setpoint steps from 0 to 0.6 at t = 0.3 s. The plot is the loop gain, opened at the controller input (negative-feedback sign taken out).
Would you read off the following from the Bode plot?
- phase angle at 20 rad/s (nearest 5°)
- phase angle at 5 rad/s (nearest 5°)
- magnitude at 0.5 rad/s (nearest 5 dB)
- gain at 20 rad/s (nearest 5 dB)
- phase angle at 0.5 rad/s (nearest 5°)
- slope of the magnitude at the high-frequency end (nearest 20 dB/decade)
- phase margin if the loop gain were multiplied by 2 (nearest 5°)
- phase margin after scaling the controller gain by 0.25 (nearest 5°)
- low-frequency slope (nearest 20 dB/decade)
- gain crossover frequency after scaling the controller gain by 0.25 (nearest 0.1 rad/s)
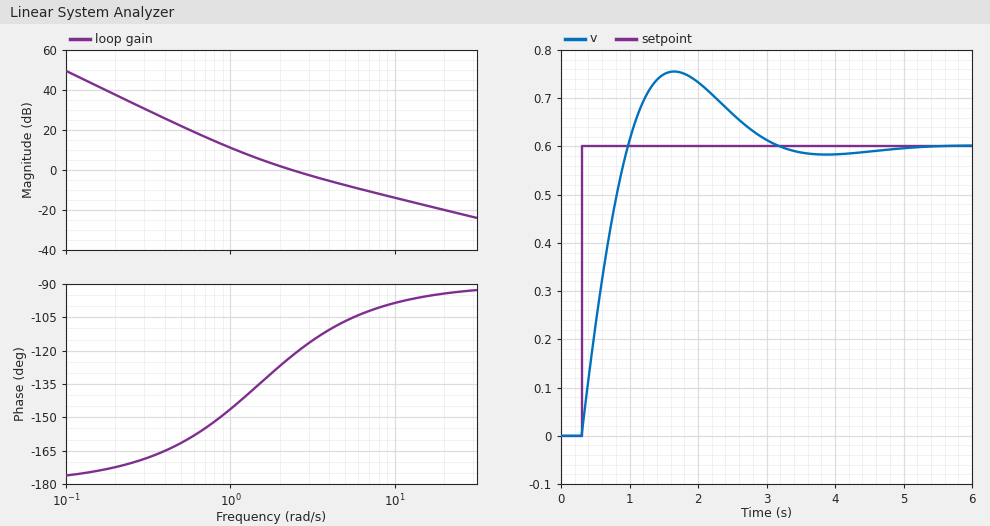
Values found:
-95°
-105°
20 dB
-20 dB
-160°
-20 dB/decade
70°
30°
-40 dB/decade
0.9 rad/s
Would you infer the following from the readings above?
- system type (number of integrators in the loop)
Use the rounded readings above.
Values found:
2
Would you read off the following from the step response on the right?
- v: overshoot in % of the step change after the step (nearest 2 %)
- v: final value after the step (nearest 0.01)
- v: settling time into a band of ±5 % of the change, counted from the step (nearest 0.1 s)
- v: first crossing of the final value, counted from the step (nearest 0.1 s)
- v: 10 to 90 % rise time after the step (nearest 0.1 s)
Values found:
26 %
0.60
2.5 s
0.7 s
0.5 s
